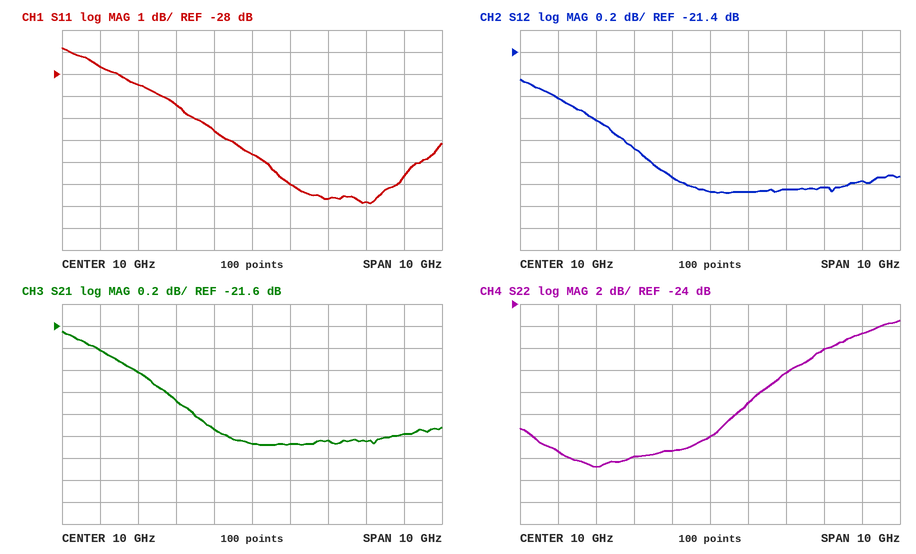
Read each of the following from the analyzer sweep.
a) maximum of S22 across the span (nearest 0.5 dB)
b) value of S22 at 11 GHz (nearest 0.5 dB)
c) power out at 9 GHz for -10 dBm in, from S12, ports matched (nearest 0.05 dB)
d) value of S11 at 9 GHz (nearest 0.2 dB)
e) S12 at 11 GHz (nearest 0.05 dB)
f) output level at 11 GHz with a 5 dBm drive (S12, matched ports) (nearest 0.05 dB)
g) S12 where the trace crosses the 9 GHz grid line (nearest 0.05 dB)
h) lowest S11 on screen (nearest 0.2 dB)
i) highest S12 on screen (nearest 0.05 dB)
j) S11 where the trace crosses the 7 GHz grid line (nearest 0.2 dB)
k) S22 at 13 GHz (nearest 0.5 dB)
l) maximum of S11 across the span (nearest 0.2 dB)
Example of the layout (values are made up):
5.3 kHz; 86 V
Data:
-25.5 dB; -33.0 dB; -32.55 dBm; -30.6 dB; -22.65 dB; -17.65 dBm; -22.55 dB; -33.8 dB; -21.65 dB; -28.4 dB; -28.0 dB; -26.8 dB
